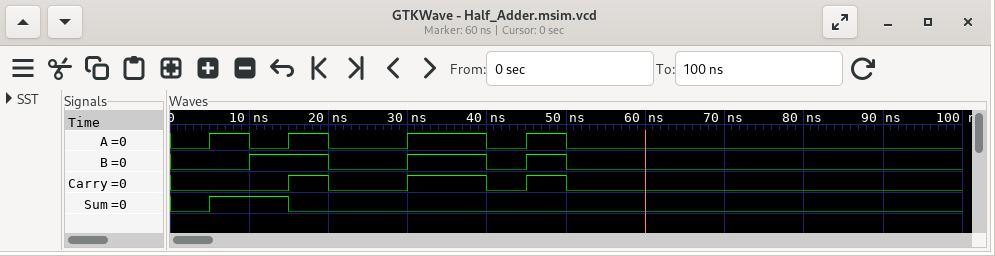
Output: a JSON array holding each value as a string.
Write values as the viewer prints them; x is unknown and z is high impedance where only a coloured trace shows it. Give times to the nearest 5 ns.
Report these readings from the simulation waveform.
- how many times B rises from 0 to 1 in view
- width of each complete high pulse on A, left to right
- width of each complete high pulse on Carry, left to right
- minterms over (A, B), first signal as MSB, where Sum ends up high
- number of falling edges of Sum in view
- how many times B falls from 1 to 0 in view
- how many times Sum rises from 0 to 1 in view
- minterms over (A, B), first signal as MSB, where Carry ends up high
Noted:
["3", "5 ns, 5 ns, 10 ns, 5 ns", "5 ns, 10 ns, 5 ns", "1, 2", "1", "3", "1", "3"]
